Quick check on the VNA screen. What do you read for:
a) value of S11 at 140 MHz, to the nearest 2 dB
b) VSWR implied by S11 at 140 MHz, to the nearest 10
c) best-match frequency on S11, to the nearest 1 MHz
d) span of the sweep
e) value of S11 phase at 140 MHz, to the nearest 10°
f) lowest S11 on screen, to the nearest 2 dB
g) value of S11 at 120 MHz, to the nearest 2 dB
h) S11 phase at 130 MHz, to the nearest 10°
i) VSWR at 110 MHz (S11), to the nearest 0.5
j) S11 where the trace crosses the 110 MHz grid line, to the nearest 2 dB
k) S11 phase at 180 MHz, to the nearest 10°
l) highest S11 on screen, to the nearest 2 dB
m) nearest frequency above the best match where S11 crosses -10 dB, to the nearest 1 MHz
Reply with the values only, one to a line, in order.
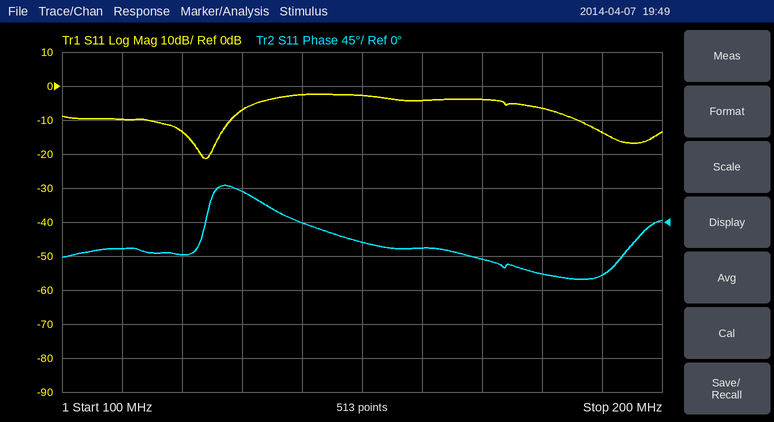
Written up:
-2 dB
10
124 MHz
100 MHz
0°
-22 dB
-14 dB
40°
2.0
-10 dB
-70°
-2 dB
128 MHz
